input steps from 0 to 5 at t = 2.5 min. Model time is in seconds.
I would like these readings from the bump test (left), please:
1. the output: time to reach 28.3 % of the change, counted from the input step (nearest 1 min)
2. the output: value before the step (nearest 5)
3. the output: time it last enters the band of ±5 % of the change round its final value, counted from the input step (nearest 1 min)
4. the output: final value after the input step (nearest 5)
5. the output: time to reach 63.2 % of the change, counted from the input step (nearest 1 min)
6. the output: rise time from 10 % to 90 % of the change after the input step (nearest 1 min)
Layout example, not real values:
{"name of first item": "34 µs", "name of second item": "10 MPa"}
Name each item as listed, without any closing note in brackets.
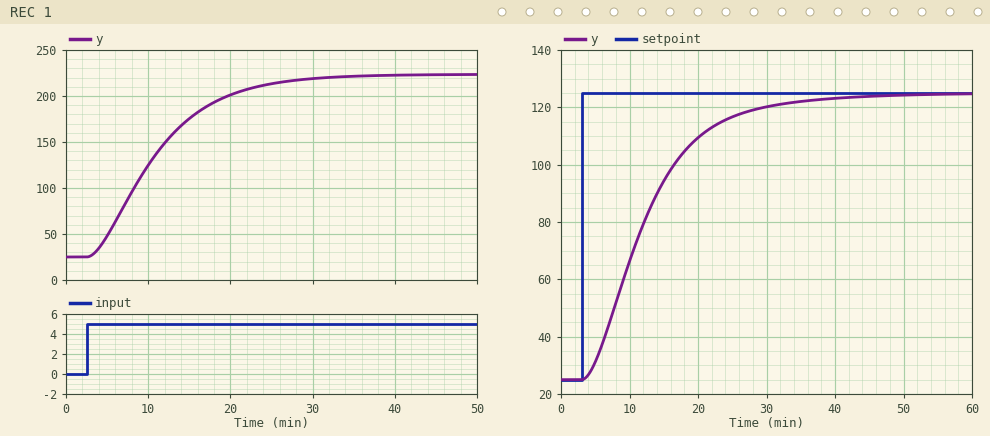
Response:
{"the output: time to reach 28.3 % of the change, counted from the input step": "5 min", "the output: value before the step": "25", "the output: time it last enters the band of ±5 % of the change round its final value, counted from the input step": "23 min", "the output: final value after the input step": "225", "the output: time to reach 63.2 % of the change, counted from the input step": "10 min", "the output: rise time from 10 % to 90 % of the change after the input step": "16 min"}
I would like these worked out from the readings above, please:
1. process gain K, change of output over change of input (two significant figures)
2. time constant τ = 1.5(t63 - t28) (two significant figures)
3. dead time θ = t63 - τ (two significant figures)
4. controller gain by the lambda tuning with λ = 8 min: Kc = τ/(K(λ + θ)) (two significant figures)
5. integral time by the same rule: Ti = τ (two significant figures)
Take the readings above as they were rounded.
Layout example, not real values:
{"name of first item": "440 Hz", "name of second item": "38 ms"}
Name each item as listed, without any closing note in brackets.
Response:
{"process gain K, change of output over change of input": "40", "time constant τ = 1.5(t63 - t28)": "7.5 min", "dead time θ = t63 - τ": "2.5 min", "controller gain by the lambda tuning with λ = 8 min: Kc = τ/(K(λ + θ))": "0.018", "integral time by the same rule: Ti = τ": "7.5 min"}
